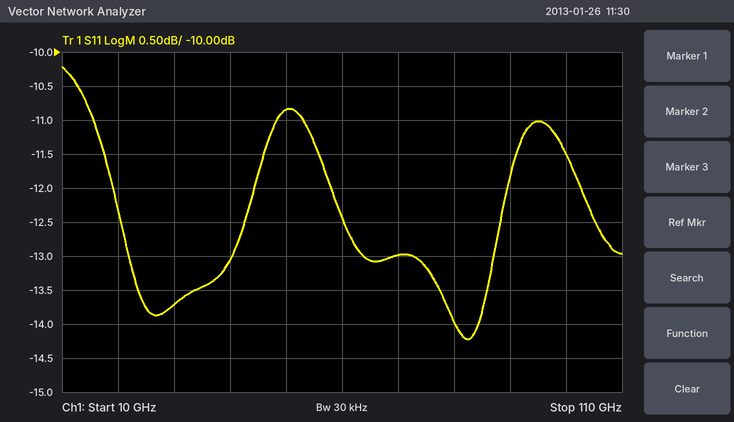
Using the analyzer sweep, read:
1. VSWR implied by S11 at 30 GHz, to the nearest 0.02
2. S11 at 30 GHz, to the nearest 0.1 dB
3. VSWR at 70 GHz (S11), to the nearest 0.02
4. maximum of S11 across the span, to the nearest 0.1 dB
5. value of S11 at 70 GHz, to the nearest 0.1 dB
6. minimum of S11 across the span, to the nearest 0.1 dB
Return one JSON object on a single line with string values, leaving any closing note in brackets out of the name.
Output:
{"VSWR implied by S11 at 30 GHz, to the nearest 0.02": "1.52", "S11 at 30 GHz, to the nearest 0.1 dB": "-13.7 dB", "VSWR at 70 GHz (S11), to the nearest 0.02": "1.58", "maximum of S11 across the span, to the nearest 0.1 dB": "-10.2 dB", "value of S11 at 70 GHz, to the nearest 0.1 dB": "-13.0 dB", "minimum of S11 across the span, to the nearest 0.1 dB": "-14.2 dB"}
